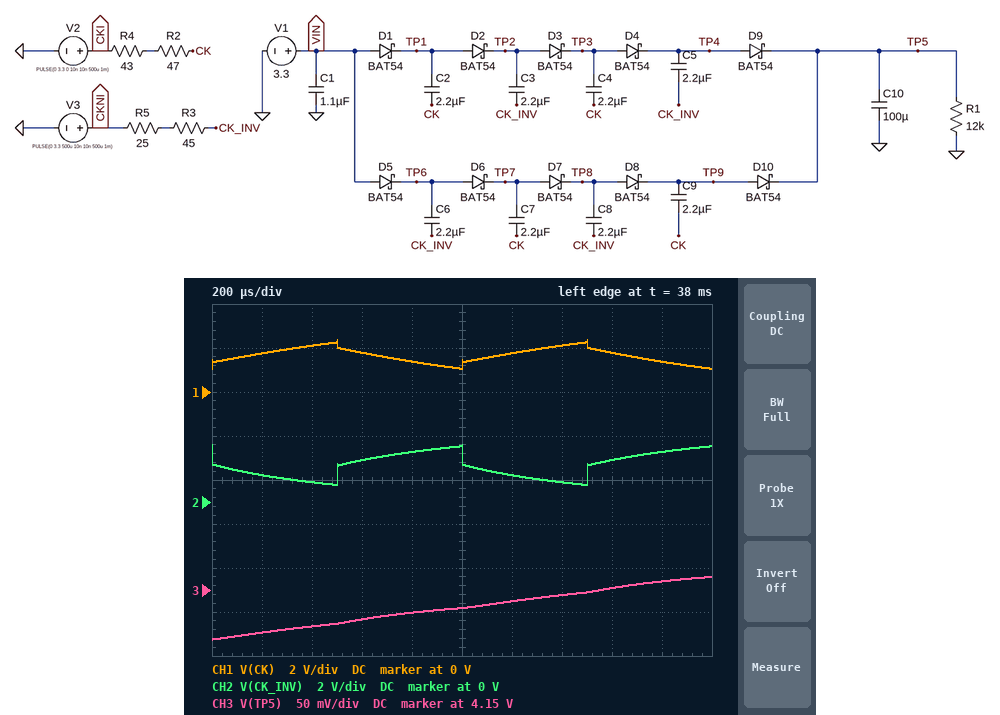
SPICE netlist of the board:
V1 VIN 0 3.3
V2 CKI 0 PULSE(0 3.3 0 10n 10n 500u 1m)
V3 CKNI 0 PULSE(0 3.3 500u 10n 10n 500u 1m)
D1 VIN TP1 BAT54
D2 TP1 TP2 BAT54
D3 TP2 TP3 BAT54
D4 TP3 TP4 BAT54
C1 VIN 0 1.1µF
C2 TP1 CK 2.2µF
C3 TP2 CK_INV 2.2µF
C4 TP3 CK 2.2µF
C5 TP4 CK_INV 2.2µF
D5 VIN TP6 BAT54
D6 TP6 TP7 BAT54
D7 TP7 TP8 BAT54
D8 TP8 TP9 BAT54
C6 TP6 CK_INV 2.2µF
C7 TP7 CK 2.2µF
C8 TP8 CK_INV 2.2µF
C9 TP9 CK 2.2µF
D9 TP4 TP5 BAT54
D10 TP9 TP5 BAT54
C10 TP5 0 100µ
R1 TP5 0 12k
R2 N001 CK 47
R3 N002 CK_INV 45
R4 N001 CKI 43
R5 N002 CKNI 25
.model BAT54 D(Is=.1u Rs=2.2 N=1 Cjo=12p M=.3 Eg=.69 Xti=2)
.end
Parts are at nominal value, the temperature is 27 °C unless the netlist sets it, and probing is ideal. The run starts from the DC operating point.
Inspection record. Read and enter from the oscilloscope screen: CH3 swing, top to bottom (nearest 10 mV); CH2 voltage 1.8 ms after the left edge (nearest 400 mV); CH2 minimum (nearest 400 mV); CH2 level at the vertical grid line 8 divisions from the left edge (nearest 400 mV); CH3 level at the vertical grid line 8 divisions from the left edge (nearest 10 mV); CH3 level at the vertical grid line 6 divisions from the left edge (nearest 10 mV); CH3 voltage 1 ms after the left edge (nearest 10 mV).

70 mV
2.4 V
800 mV
2.0 V
4.15 V
4.14 V
4.13 V
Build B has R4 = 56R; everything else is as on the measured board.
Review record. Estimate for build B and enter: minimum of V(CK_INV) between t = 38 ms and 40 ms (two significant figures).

740 mV
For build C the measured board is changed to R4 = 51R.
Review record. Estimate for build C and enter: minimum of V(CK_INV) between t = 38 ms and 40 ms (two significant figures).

750 mV
